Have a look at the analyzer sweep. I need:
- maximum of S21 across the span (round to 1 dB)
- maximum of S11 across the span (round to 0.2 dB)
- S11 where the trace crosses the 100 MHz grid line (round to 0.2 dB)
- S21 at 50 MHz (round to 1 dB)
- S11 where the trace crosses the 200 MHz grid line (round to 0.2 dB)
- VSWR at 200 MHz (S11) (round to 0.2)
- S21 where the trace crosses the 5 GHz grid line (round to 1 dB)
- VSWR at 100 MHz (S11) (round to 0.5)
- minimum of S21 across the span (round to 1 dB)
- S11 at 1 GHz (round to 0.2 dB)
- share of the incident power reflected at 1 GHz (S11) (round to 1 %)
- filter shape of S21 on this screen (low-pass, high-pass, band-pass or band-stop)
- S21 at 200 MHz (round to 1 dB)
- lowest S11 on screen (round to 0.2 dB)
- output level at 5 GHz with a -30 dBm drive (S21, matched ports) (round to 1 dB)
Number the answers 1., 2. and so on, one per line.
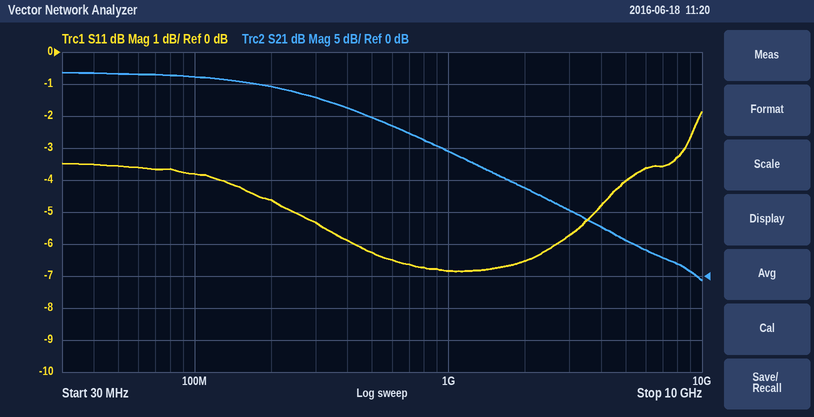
1. 32 dB
2. -1.8 dB
3. -3.8 dB
4. 32 dB
5. -4.6 dB
6. 3.8
7. 6 dB
8. 4.5
9. -1 dB
10. -6.8 dB
11. 21 %
12. low-pass
13. 30 dB
14. -6.8 dB
15. -24 dBm
